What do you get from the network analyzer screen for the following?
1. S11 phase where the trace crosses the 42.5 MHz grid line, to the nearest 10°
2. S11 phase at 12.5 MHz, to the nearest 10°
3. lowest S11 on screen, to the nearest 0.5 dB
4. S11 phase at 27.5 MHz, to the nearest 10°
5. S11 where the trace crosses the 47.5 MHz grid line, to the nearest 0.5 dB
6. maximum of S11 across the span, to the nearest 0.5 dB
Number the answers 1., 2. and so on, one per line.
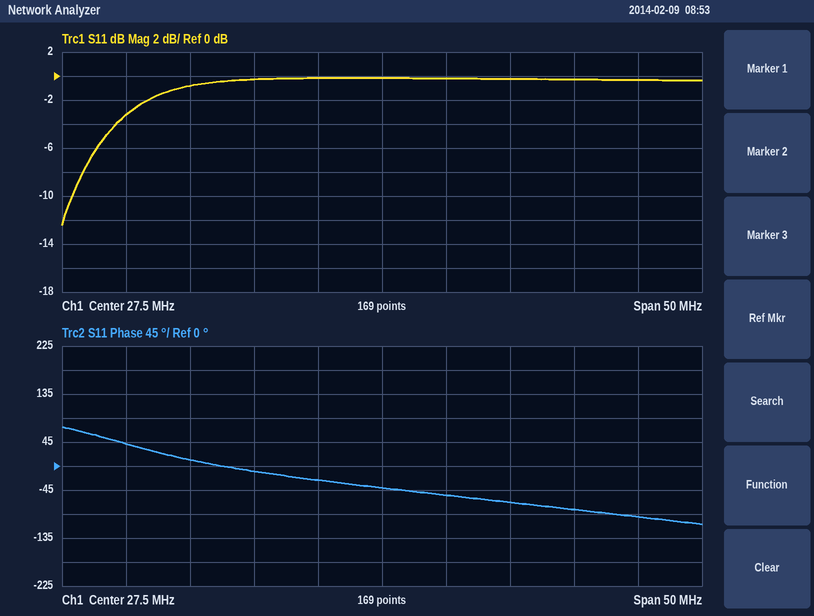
1. -80°
2. 10°
3. -12.5 dB
4. -40°
5. -0.5 dB
6. 0.0 dB
